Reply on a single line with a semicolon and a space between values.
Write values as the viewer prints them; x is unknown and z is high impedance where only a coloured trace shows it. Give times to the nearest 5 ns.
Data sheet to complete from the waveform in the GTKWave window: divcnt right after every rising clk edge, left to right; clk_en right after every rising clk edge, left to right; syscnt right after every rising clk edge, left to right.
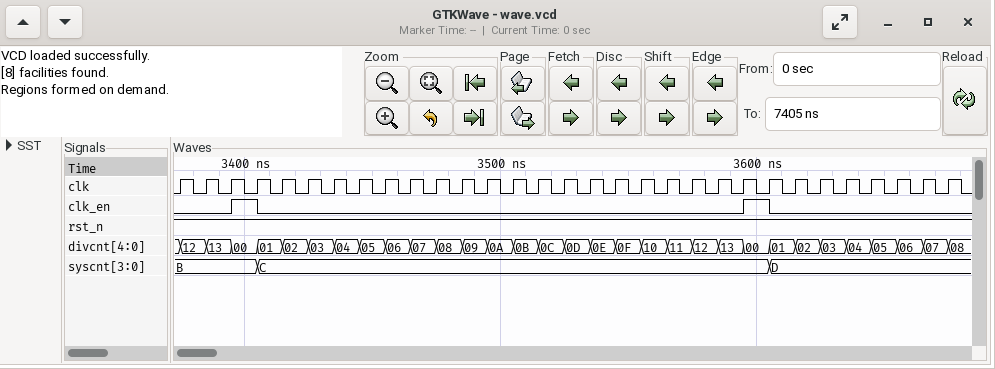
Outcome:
12, 13, 00, 01, 02, 03, 04, 05, 06, 07, 08, 09, 0A, 0B, 0C, 0D, 0E, 0F, 10, 11, 12, 13, 00, 01, 02, 03, 04, 05, 06, 07, 08; 0 0 1 0 0 0 0 0 0 0 0 0 0 0 0 0 0 0 0 0 0 0 1 0 0 0 0 0 0 0 0; B, B, B, C, C, C, C, C, C, C, C, C, C, C, C, C, C, C, C, C, C, C, C, D, D, D, D, D, D, D, D
